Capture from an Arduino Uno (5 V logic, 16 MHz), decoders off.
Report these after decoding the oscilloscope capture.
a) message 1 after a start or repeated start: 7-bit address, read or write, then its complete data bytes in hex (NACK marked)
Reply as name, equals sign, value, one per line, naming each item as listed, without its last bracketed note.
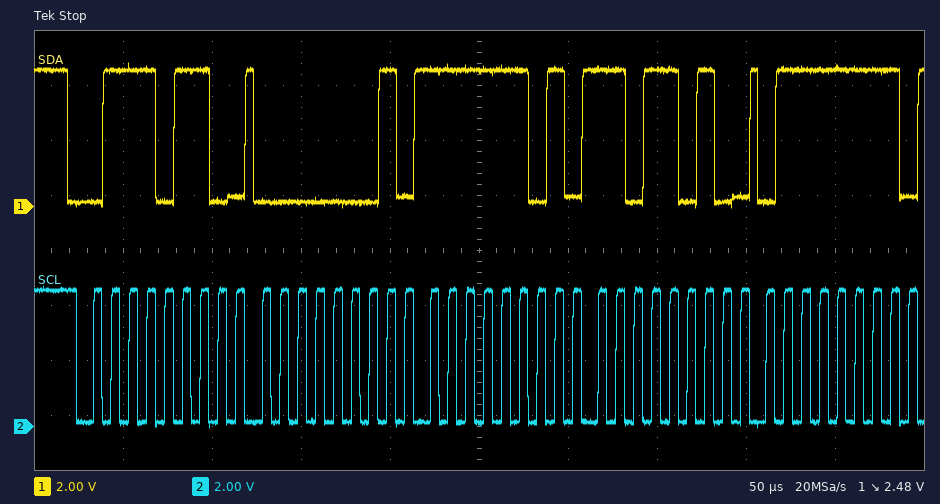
message 1 after a start or repeated start: 7-bit address, read or write, then its complete data bytes in hex = 0x3B write: 01 FD DA 7F
